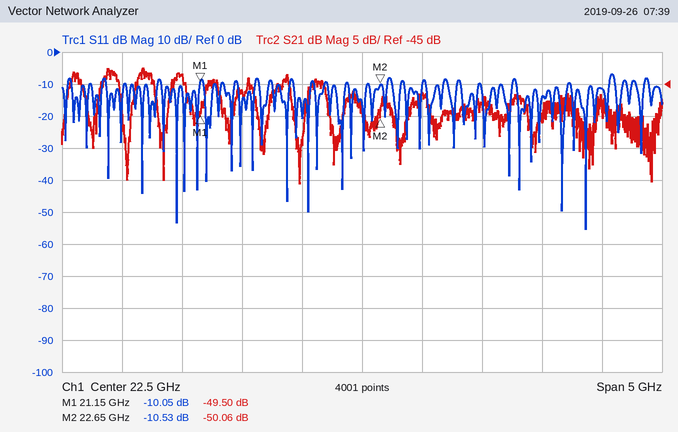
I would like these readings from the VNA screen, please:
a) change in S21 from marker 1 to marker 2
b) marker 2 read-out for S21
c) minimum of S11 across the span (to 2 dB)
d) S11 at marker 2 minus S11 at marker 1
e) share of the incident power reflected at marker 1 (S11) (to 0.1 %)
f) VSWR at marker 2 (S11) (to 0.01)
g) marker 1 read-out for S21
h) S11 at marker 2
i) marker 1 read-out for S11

-0.56 dB
-50.06 dB
-56 dB
-0.48 dB
9.9 %
1.85
-49.50 dB
-10.53 dB
-10.05 dB
